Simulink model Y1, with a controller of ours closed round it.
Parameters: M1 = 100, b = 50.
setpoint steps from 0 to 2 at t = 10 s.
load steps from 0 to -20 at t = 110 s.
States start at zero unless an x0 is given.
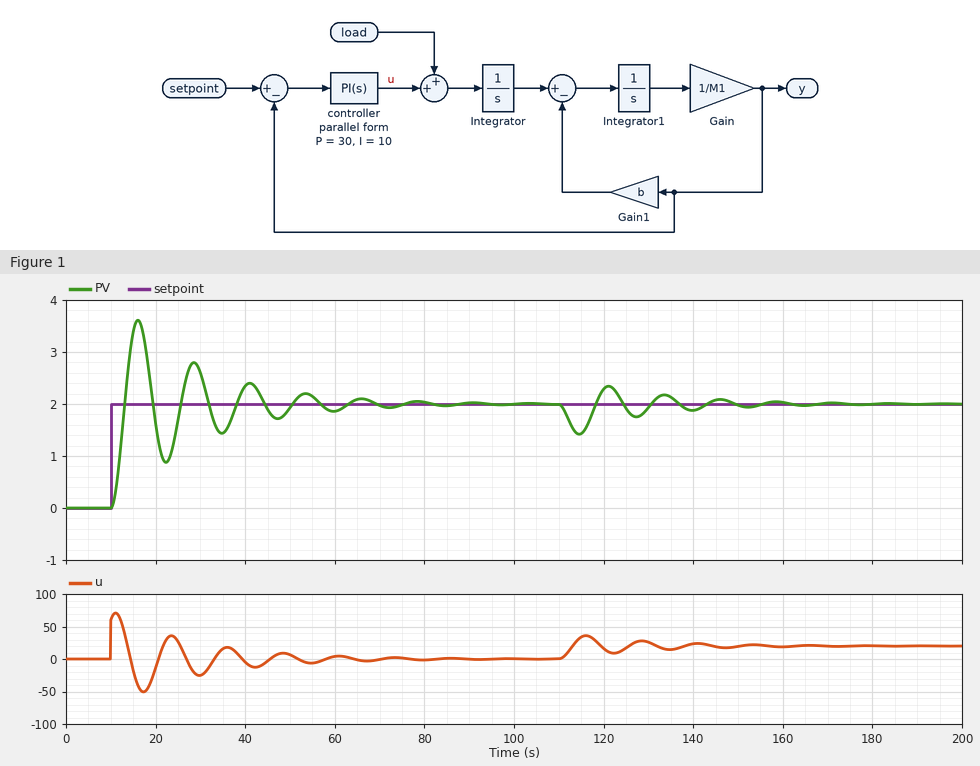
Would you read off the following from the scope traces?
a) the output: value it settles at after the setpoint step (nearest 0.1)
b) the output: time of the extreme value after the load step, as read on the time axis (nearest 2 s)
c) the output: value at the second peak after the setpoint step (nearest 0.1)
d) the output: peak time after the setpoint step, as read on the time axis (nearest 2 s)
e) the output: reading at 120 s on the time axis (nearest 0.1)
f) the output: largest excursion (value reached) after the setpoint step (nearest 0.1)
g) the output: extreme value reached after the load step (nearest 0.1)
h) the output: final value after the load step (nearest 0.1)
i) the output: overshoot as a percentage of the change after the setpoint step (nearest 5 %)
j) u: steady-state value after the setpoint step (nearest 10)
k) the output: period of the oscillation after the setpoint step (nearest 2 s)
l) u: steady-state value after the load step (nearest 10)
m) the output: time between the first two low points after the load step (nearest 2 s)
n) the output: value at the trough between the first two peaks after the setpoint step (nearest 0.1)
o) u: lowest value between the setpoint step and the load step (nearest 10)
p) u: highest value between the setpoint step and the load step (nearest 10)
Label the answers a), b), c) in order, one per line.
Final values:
a) 2.0
b) 114 s
c) 2.8
d) 16 s
e) 2.3
f) 3.6
g) 1.4
h) 2.0
i) 80 %
j) 0
k) 12 s
l) 20
m) 12 s
n) 0.9
o) -50
p) 70
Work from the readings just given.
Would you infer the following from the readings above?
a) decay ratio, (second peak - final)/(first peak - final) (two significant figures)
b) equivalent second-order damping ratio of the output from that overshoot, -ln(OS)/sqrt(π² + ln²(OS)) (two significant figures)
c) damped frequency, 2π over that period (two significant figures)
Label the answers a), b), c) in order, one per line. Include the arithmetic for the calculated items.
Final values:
a) (2.8 - 2) / (3.6 - 2) = 0.50
b) ln(0.8) = -0.223; 0.223 / sqrt(9.870 + 0.050) = 0.071
c) 2π / 12 = 0.52 rad/s
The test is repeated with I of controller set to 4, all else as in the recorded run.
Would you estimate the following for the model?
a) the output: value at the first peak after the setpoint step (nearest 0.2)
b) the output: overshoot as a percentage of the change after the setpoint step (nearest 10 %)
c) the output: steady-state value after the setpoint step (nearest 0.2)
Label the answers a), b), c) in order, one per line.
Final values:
a) 3.0
b) 50 %
c) 2.0
